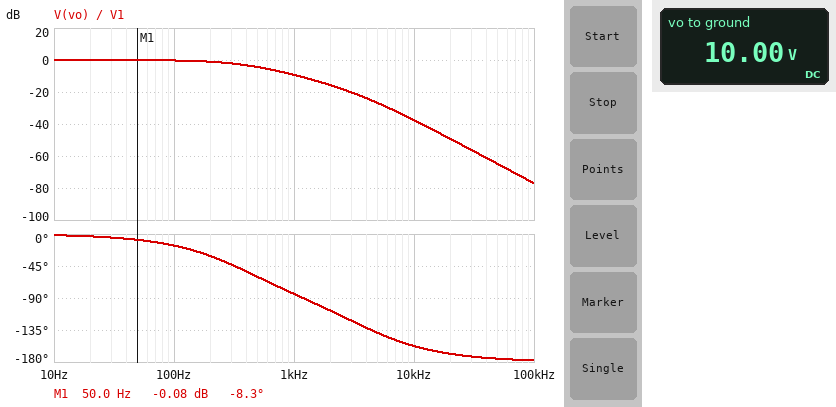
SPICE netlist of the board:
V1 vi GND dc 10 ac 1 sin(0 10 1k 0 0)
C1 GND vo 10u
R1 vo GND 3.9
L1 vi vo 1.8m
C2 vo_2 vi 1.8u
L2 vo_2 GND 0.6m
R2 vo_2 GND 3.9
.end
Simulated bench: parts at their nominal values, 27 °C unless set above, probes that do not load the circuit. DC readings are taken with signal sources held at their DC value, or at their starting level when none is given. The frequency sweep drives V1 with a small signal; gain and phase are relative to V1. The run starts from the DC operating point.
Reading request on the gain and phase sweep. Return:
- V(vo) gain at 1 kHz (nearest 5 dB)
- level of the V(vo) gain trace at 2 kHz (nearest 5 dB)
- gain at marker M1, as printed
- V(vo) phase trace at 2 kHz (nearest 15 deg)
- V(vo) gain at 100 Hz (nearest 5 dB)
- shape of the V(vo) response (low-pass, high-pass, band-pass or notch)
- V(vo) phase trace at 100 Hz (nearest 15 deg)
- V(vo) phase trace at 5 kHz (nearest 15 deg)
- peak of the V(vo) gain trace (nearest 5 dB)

-10 dB
-15 dB
-0.08 dB
-105 deg
0 dB
low-pass
-15 deg
-135 deg
0 dB
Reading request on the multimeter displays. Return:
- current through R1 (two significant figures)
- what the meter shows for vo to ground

2.6 A
10.00 V
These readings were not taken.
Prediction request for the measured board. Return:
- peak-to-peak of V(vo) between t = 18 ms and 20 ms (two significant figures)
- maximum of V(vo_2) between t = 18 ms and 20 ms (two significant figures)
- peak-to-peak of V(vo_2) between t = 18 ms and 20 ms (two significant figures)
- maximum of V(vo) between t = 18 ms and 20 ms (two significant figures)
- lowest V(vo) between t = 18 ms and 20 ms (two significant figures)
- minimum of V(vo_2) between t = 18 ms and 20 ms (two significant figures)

6.9 V
310 mV
630 mV
3.4 V
-3.4 V
-310 mV
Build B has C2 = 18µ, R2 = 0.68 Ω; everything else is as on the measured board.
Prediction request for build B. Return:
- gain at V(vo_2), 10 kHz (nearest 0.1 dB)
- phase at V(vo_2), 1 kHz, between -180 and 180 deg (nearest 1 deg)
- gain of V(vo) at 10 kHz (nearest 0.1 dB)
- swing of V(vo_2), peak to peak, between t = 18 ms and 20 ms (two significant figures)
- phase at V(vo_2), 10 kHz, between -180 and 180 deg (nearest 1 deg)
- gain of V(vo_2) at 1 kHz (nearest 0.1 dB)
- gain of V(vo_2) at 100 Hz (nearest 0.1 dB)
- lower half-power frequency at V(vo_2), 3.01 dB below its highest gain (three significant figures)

-4.2 dB
96 deg
-37.6 dB
1.5 V
53 deg
-22.3 dB
-48.5 dB
12.8 kHz
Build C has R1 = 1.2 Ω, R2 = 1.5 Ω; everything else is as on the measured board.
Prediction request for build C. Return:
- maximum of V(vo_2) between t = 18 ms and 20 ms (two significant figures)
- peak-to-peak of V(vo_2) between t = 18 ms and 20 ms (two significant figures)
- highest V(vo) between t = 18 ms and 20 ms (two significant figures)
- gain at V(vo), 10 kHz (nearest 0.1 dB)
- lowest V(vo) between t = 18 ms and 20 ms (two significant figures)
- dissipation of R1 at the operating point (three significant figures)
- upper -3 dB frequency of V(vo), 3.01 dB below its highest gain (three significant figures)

160 mV
320 mV
1.1 V
-41.4 dB
-1.1 V
83.3 W
107 Hz
